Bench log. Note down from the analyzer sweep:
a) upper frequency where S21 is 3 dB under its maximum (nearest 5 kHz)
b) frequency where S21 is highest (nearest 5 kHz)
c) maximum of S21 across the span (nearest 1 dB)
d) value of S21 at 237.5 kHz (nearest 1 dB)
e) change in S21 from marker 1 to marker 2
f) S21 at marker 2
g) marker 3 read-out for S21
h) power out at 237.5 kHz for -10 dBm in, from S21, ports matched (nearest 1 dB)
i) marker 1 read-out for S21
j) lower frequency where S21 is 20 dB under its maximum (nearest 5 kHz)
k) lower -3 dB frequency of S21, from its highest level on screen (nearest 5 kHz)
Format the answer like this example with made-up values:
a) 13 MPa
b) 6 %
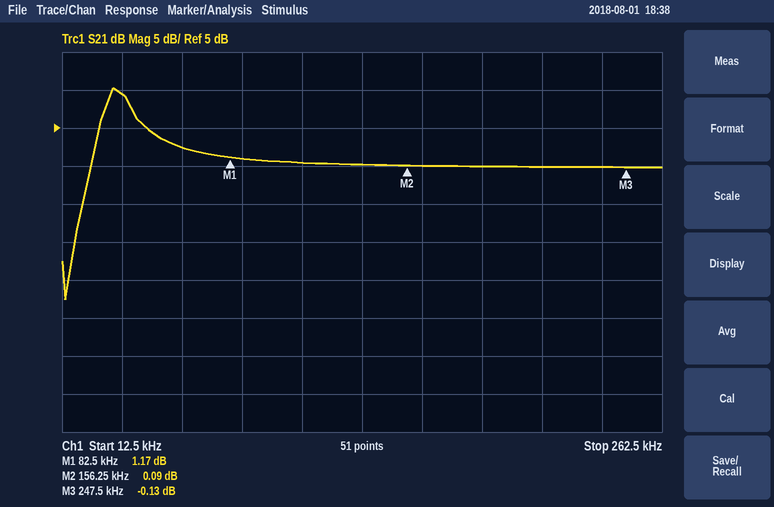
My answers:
a) 40 kHz
b) 35 kHz
c) 10 dB
d) 0 dB
e) -1.08 dB
f) 0.09 dB
g) -0.13 dB
h) -10 dBm
i) 1.17 dB
j) 20 kHz
k) 30 kHz
